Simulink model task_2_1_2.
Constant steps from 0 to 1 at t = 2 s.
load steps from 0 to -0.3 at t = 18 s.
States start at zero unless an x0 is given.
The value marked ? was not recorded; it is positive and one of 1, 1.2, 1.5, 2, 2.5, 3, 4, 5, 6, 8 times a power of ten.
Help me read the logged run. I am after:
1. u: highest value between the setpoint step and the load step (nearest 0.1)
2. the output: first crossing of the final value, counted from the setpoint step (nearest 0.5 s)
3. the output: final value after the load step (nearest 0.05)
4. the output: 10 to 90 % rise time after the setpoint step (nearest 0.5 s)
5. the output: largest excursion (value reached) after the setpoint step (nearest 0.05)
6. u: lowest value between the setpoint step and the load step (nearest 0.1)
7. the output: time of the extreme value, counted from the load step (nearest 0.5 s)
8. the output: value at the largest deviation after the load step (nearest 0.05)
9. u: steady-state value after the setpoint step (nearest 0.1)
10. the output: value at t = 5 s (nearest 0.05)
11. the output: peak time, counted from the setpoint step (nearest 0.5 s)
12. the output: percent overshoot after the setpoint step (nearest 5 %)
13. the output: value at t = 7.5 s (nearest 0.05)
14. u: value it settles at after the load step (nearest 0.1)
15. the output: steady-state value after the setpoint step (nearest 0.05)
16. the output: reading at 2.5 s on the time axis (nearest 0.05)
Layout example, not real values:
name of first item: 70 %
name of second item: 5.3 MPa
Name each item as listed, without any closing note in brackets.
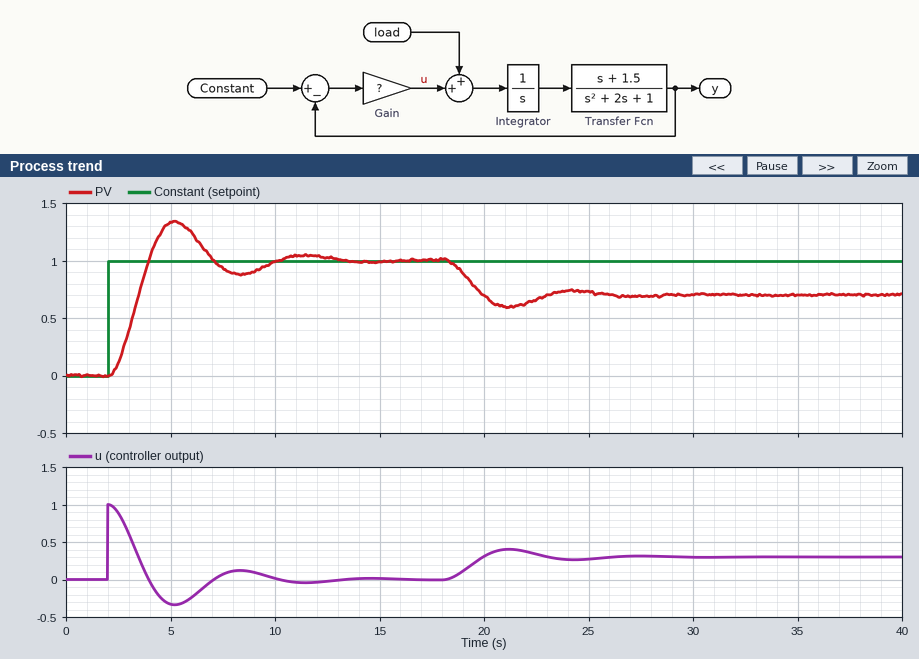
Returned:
u: highest value between the setpoint step and the load step: 1.0
the output: first crossing of the final value, counted from the setpoint step: 2.0 s
the output: final value after the load step: 0.70
the output: 10 to 90 % rise time after the setpoint step: 1.5 s
the output: largest excursion (value reached) after the setpoint step: 1.35
u: lowest value between the setpoint step and the load step: -0.3
the output: time of the extreme value, counted from the load step: 3.0 s
the output: value at the largest deviation after the load step: 0.60
u: steady-state value after the setpoint step: 0.0
the output: value at t = 5 s: 1.35
the output: peak time, counted from the setpoint step: 3.0 s
the output: percent overshoot after the setpoint step: 35 %
the output: value at t = 7.5 s: 0.95
u: value it settles at after the load step: 0.3
the output: steady-state value after the setpoint step: 1.00
the output: reading at 2.5 s on the time axis: 0.10
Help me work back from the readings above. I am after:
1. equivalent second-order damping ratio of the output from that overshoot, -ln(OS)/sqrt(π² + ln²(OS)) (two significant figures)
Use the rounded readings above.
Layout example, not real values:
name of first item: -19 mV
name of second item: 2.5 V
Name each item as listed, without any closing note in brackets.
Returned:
equivalent second-order damping ratio of the output from that overshoot, -ln(OS)/sqrt(π² + ln²(OS)): 0.32
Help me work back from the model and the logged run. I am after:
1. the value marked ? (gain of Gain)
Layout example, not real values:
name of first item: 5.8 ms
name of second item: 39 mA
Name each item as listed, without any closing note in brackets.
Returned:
the value marked ?: 1
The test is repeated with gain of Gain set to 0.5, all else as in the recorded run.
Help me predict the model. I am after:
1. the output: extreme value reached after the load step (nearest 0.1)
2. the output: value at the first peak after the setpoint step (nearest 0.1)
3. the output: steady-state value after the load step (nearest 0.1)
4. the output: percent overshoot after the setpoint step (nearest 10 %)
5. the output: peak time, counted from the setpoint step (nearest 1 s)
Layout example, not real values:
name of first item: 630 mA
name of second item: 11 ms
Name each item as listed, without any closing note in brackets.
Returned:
the output: extreme value reached after the load step: 0.3
the output: value at the first peak after the setpoint step: 1.2
the output: steady-state value after the load step: 0.4
the output: percent overshoot after the setpoint step: 20 %
the output: peak time, counted from the setpoint step: 5 s
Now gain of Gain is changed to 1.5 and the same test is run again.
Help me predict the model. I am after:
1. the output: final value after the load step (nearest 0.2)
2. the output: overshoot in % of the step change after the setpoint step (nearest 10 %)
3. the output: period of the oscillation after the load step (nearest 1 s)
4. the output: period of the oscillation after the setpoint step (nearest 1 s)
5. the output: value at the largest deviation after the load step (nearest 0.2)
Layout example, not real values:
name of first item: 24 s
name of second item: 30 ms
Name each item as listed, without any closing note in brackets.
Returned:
the output: final value after the load step: 0.8
the output: overshoot in % of the step change after the setpoint step: 40 %
the output: period of the oscillation after the load step: 5 s
the output: period of the oscillation after the setpoint step: 5 s
the output: value at the largest deviation after the load step: 0.8
